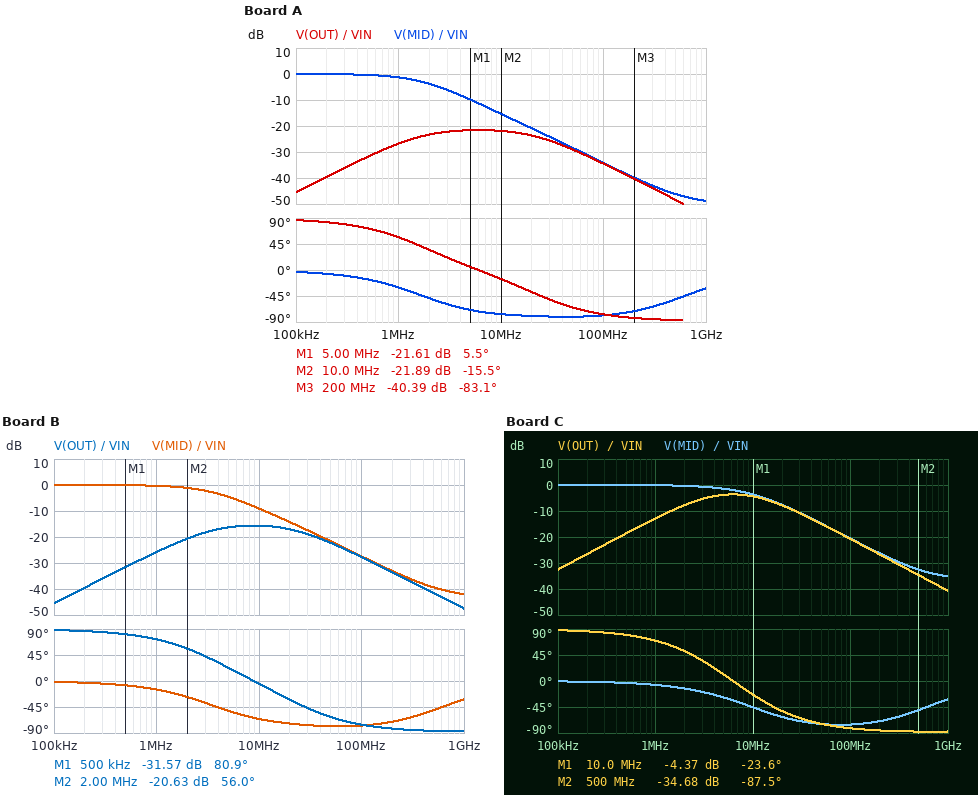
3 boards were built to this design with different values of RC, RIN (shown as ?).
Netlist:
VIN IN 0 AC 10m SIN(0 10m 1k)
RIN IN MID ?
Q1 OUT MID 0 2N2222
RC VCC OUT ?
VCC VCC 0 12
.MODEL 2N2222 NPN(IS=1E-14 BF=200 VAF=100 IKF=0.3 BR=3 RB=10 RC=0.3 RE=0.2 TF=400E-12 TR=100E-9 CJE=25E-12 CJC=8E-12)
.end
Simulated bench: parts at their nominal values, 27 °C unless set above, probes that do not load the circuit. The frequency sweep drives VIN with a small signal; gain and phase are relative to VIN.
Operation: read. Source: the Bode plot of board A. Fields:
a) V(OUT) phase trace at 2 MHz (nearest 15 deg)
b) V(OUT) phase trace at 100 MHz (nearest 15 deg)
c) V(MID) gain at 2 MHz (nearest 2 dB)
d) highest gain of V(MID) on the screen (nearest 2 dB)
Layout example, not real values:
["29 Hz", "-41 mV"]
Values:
["30 deg", "-75 deg", "-4 dB", "0 dB"]
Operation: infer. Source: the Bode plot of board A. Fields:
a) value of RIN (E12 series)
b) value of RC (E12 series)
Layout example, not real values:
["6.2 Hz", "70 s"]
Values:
["3.3 kΩ", "2.7 kΩ"]
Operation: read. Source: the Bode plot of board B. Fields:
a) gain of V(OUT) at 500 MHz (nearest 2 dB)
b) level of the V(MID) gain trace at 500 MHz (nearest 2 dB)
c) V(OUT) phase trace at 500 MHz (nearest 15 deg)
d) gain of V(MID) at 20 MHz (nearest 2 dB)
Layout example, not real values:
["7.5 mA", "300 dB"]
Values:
["-42 dB", "-40 dB", "-90 deg", "-14 dB"]
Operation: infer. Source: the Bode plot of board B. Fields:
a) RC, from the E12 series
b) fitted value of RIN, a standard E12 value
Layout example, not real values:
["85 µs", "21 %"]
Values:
["2.7 kΩ", "1.5 kΩ"]
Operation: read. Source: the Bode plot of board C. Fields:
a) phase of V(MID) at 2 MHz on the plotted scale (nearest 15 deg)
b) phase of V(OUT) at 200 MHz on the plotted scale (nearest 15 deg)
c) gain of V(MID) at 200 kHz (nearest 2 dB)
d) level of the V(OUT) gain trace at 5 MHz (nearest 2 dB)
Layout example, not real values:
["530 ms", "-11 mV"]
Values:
["-15 deg", "-90 deg", "0 dB", "-4 dB"]
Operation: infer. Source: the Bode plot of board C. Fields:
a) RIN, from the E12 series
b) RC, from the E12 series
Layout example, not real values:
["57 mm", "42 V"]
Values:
["680 Ω", "12 kΩ"]
